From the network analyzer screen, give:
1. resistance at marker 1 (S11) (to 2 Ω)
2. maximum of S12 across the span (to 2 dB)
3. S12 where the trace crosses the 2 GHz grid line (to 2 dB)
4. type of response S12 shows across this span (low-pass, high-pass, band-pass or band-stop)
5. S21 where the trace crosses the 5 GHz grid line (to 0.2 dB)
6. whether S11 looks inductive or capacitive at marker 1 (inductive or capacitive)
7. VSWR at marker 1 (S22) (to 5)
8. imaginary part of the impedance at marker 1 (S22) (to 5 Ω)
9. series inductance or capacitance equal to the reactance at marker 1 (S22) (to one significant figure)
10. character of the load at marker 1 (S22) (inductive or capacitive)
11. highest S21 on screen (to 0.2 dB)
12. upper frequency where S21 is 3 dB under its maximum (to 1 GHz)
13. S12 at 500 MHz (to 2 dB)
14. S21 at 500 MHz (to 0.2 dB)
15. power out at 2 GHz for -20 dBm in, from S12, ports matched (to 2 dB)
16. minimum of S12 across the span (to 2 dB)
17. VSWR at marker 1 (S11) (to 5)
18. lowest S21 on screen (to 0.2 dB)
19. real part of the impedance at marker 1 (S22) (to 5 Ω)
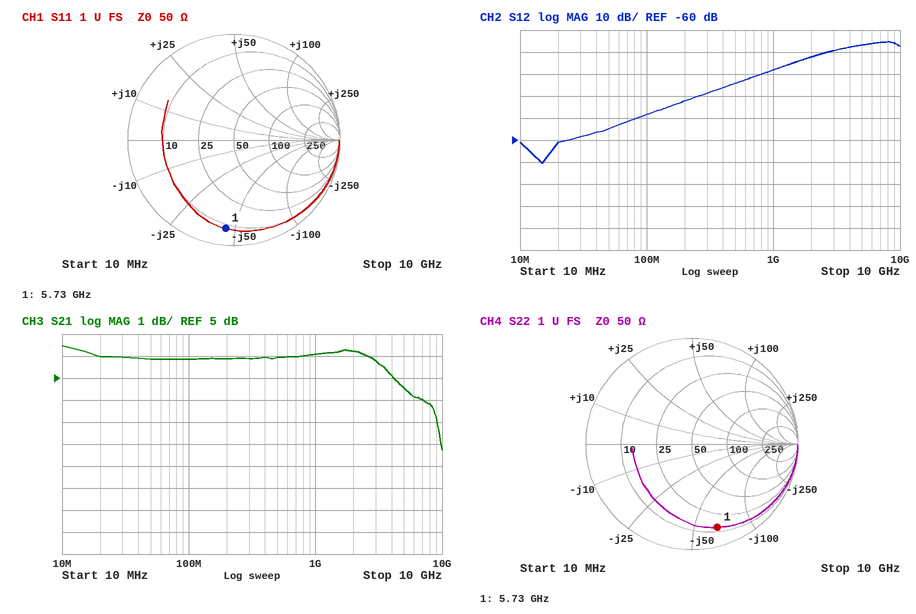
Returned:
8 Ω
-16 dB
-22 dB
high-pass
4.6 dB
capacitive
10
-65 Ω
400 fF
capacitive
6.4 dB
9 GHz
-34 dB
6.0 dB
-42 dBm
-70 dB
10
1.8 dB
15 Ω
